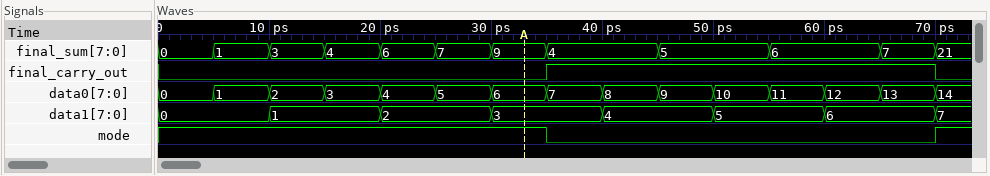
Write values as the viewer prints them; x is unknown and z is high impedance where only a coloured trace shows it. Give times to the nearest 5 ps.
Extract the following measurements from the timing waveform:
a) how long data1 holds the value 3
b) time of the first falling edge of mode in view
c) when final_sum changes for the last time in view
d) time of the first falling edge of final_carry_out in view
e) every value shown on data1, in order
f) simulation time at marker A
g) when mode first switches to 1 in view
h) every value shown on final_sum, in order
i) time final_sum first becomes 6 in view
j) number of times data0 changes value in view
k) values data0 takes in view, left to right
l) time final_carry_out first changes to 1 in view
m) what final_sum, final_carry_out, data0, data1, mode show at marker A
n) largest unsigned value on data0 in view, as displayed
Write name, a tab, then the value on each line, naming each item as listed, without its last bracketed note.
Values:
how long data1 holds the value 3	10 ps
time of the first falling edge of mode in view	35 ps
when final_sum changes for the last time in view	70 ps
time of the first falling edge of final_carry_out in view	70 ps
every value shown on data1, in order	0, 1, 2, 3, 4, 5, 6, 7
simulation time at marker A	35 ps
when mode first switches to 1 in view	70 ps
every value shown on final_sum, in order	0, 1, 3, 4, 6, 7, 9, 4, 5, 6, 7, 21
time final_sum first becomes 6 in view	20 ps
number of times data0 changes value in view	14
values data0 takes in view, left to right	0, 1, 2, 3, 4, 5, 6, 7, 8, 9, 10, 11, 12, 13, 14
time final_carry_out first changes to 1 in view	35 ps
what final_sum, final_carry_out, data0, data1, mode show at marker A	final_sum=9, final_carry_out=0, data0=6, data1=3, mode=1
largest unsigned value on data0 in view, as displayed	14
